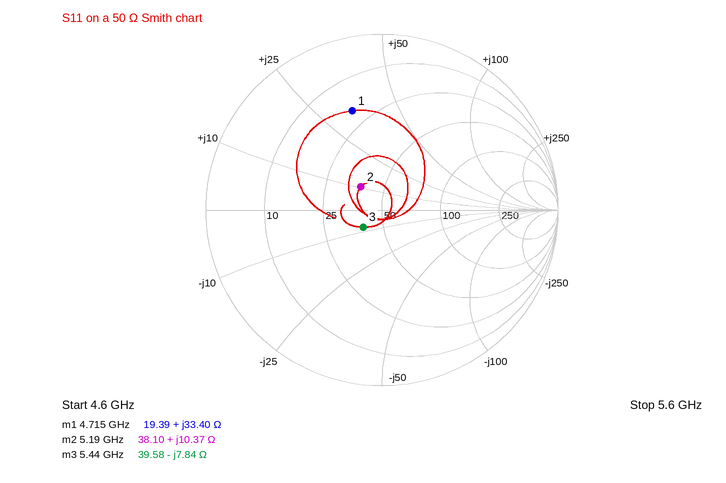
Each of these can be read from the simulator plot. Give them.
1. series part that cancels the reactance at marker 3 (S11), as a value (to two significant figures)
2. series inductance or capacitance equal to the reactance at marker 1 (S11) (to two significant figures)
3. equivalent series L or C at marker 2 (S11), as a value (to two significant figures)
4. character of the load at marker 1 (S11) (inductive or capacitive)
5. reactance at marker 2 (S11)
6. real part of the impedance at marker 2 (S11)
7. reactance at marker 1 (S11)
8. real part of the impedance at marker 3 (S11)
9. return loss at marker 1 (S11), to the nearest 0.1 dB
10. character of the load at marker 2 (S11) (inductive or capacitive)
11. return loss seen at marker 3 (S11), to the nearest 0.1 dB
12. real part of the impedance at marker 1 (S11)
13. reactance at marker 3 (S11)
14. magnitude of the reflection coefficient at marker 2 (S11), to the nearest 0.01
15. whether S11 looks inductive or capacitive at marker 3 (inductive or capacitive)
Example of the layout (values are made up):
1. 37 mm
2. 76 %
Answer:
1. 230 pH
2. 1.1 nH
3. 320 pH
4. inductive
5. +10.37 Ω
6. 38.10 Ω
7. +33.40 Ω
8. 39.58 Ω
9. 4.6 dB
10. inductive
11. 16.8 dB
12. 19.39 Ω
13. -7.84 Ω
14. 0.18
15. capacitive
